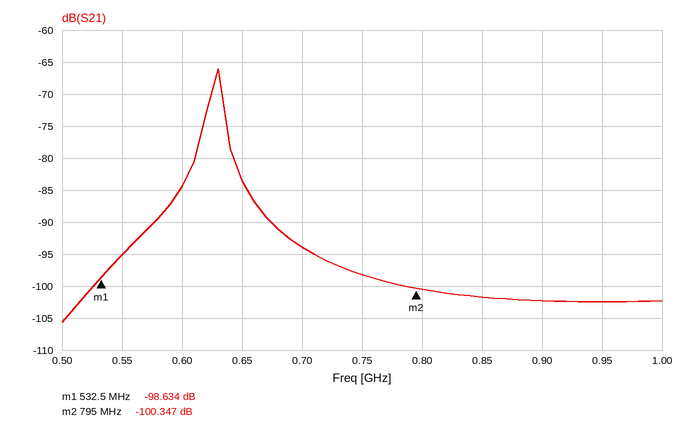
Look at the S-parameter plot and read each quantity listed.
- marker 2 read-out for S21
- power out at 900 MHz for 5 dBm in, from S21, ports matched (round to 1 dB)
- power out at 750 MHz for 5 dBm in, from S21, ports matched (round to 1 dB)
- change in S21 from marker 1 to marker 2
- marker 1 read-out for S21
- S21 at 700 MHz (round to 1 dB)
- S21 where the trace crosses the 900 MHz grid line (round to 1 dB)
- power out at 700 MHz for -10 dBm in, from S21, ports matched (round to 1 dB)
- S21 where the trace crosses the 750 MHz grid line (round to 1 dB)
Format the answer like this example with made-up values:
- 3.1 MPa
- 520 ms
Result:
- -100.347 dB
- -97 dBm
- -93 dBm
- -1.713 dB
- -98.634 dB
- -94 dB
- -102 dB
- -104 dBm
- -98 dB
